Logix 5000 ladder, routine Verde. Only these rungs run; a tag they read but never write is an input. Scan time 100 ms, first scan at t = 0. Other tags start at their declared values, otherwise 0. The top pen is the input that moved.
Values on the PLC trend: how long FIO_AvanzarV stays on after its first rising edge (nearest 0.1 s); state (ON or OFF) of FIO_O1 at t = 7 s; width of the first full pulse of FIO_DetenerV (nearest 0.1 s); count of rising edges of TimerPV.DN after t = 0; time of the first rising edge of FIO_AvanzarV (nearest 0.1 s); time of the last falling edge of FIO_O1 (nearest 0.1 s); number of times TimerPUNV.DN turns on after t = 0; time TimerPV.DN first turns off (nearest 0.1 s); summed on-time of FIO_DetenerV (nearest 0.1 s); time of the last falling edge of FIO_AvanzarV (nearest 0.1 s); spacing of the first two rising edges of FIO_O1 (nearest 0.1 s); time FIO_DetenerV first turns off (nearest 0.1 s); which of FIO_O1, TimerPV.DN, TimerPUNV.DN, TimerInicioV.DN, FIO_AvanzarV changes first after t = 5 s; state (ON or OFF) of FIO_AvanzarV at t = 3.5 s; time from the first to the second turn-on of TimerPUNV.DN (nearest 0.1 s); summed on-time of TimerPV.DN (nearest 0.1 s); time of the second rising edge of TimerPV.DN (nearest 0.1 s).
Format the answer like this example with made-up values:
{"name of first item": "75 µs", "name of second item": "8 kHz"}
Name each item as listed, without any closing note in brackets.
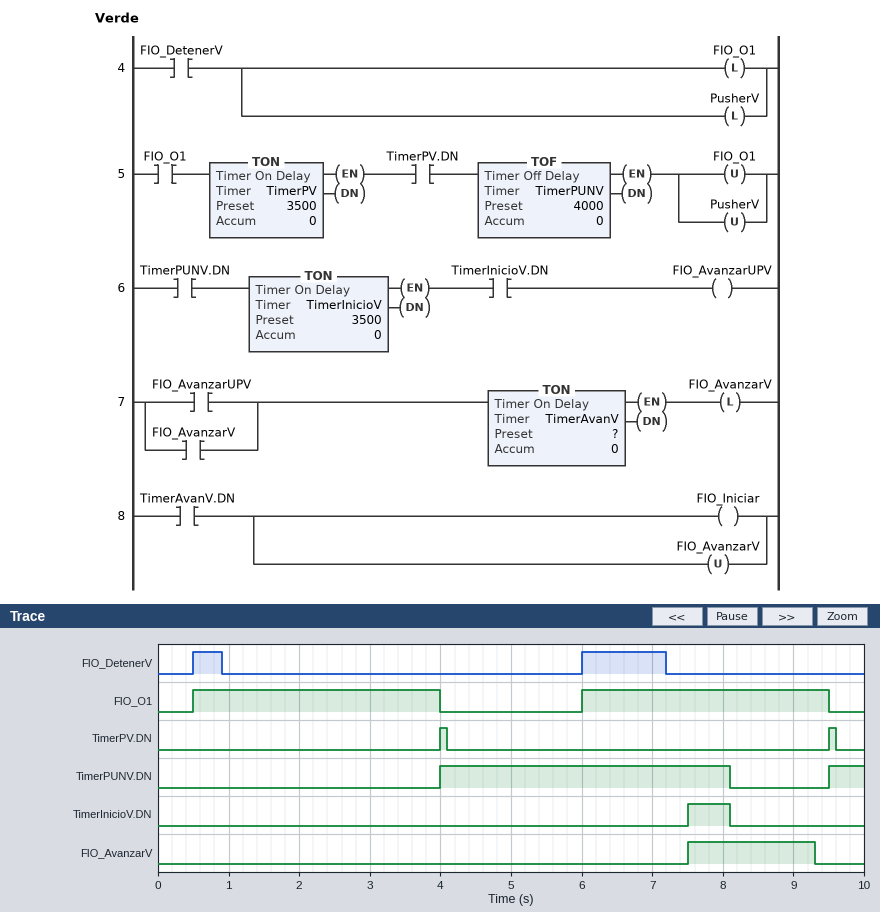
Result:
{"how long FIO_AvanzarV stays on after its first rising edge": "1.8 s", "state (ON or OFF) of FIO_O1 at t = 7 s": "ON", "width of the first full pulse of FIO_DetenerV": "0.4 s", "count of rising edges of TimerPV.DN after t = 0": "2", "time of the first rising edge of FIO_AvanzarV": "7.5 s", "time of the last falling edge of FIO_O1": "9.5 s", "number of times TimerPUNV.DN turns on after t = 0": "2", "time TimerPV.DN first turns off": "4.1 s", "summed on-time of FIO_DetenerV": "1.6 s", "time of the last falling edge of FIO_AvanzarV": "9.3 s", "spacing of the first two rising edges of FIO_O1": "5.5 s", "time FIO_DetenerV first turns off": "0.9 s", "which of FIO_O1, TimerPV.DN, TimerPUNV.DN, TimerInicioV.DN, FIO_AvanzarV changes first after t = 5 s": "FIO_O1", "state (ON or OFF) of FIO_AvanzarV at t = 3.5 s": "OFF", "time from the first to the second turn-on of TimerPUNV.DN": "5.5 s", "summed on-time of TimerPV.DN": "0.2 s", "time of the second rising edge of TimerPV.DN": "9.5 s"}
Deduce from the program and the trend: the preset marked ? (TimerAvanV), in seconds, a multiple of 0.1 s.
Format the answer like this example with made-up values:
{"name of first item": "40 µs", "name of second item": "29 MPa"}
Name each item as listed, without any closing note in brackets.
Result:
{"the preset marked ? (TimerAvanV), in seconds, a multiple of 0.1 s": "1.8 s"}
